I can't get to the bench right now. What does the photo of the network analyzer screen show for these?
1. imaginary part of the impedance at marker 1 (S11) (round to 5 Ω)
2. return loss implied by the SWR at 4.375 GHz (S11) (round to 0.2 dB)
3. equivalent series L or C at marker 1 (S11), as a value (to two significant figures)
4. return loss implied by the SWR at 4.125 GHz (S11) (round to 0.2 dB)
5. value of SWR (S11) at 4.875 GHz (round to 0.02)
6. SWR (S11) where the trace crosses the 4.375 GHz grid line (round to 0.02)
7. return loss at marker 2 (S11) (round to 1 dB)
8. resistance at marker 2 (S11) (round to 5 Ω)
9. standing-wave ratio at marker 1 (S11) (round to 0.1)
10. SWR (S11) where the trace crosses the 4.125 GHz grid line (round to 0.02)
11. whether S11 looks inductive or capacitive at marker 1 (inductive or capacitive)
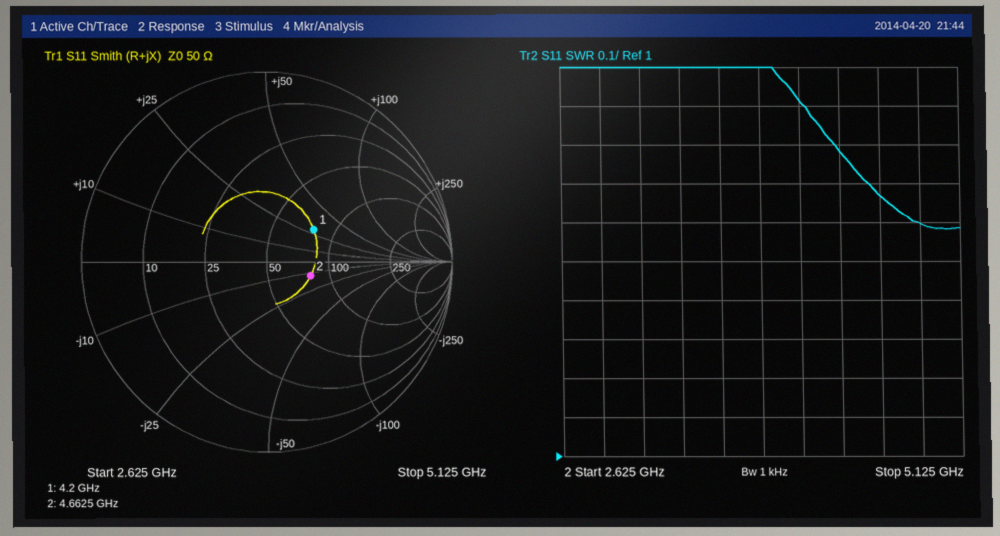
+30 Ω
11.0 dB
1.1 nH
10.0 dB
1.60
1.78
12 dB
80 Ω
1.9
1.92
inductive
